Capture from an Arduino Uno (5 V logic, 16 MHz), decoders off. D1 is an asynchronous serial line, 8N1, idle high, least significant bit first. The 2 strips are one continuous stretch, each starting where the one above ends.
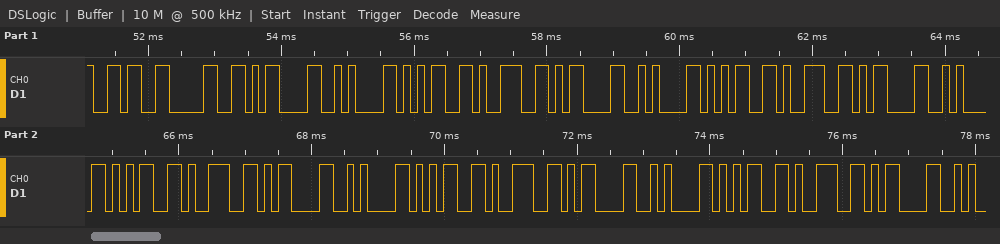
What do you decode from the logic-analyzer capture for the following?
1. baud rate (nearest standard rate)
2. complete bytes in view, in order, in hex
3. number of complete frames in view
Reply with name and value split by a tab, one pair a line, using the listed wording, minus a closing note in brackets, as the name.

baud rate	9600 baud
complete bytes in view, in order, in hex	36 30 0D 0A 35 39 0D 0A 35 39 0D 0A 35 39 0D 0A 35 39 0D 0A 35 39 0D
number of complete frames in view	23
